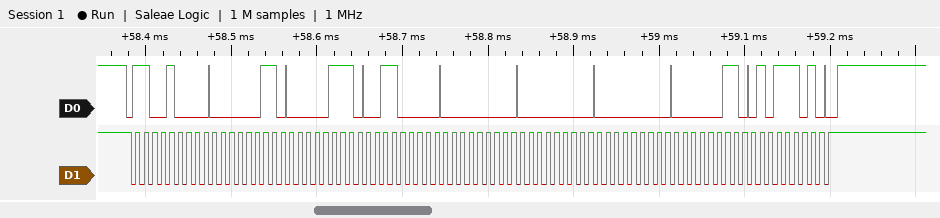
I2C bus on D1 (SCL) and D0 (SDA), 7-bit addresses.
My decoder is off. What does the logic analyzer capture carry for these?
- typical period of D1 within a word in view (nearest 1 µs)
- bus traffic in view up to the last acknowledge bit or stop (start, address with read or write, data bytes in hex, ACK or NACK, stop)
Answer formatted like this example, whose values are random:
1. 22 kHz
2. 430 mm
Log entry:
1. 10 µs
2. start, address 64 write ACK, 03 ACK, 07 ACK, 30 ACK, 00 ACK, 00 ACK, 00 ACK, 03 ACK, 5D ACK, stop
